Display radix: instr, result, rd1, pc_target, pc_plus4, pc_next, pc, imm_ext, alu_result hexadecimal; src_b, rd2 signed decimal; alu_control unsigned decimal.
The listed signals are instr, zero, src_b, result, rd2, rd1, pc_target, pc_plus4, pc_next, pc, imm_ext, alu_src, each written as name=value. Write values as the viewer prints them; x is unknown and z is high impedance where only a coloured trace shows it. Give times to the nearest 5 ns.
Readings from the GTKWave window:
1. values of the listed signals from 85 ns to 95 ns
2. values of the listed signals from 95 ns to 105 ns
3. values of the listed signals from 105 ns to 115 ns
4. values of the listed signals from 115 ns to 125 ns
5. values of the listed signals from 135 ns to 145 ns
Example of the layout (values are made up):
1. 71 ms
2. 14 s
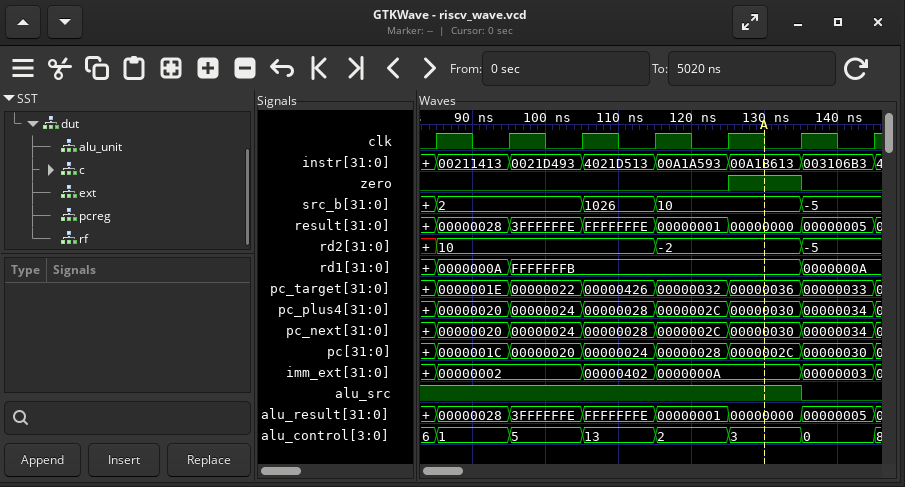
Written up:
1. instr=00211413, zero=0, src_b=2, result=00000028, rd2=10, rd1=0000000A, pc_target=0000001E, pc_plus4=00000020, pc_next=00000020, pc=0000001C, imm_ext=00000002, alu_src=1
2. instr=0021D493, zero=0, src_b=2, result=3FFFFFFE, rd2=10, rd1=FFFFFFFB, pc_target=00000022, pc_plus4=00000024, pc_next=00000024, pc=00000020, imm_ext=00000002, alu_src=1
3. instr=4021D513, zero=0, src_b=1026, result=FFFFFFFE, rd2=10, rd1=FFFFFFFB, pc_target=00000426, pc_plus4=00000028, pc_next=00000028, pc=00000024, imm_ext=00000402, alu_src=1
4. instr=00A1A593, zero=0, src_b=10, result=00000001, rd2=-2, rd1=FFFFFFFB, pc_target=00000032, pc_plus4=0000002C, pc_next=0000002C, pc=00000028, imm_ext=0000000A, alu_src=1
5. instr=003106B3, zero=0, src_b=-5, result=00000005, rd2=-5, rd1=0000000A, pc_target=00000033, pc_plus4=00000034, pc_next=00000034, pc=00000030, imm_ext=00000003, alu_src=0
